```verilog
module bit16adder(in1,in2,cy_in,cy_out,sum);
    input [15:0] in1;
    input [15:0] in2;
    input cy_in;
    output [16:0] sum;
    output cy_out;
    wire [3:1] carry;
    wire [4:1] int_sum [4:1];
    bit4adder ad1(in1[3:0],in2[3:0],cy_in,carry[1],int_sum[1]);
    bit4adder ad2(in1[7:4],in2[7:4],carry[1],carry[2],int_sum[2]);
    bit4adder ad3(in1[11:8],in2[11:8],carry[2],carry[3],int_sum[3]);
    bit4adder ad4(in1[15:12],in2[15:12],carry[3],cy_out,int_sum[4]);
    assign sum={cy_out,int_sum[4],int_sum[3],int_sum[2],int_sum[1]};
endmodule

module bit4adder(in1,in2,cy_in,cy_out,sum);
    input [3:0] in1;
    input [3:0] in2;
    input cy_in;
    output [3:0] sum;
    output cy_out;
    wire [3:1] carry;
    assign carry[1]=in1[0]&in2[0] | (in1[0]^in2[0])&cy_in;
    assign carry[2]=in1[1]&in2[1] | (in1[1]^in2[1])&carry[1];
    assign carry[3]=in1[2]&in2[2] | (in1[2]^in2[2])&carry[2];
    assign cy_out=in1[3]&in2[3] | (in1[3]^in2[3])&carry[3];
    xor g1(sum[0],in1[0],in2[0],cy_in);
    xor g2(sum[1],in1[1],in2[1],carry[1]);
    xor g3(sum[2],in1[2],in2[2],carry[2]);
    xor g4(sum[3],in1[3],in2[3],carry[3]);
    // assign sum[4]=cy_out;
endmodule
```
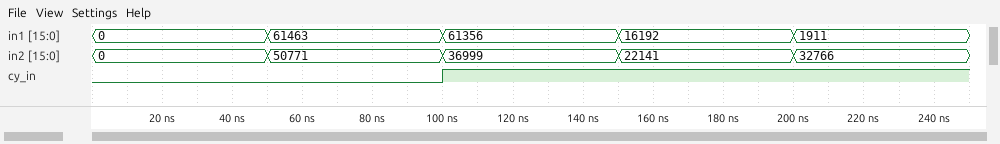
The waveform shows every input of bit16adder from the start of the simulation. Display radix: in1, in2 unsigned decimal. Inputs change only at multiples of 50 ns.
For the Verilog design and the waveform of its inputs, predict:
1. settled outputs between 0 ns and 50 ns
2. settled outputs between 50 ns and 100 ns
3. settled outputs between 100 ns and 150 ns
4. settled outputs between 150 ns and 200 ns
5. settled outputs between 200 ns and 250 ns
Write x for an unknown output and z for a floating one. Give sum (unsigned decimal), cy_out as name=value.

sum=0, cy_out=0
sum=112234, cy_out=1
sum=98356, cy_out=1
sum=38334, cy_out=0
sum=34678, cy_out=0
